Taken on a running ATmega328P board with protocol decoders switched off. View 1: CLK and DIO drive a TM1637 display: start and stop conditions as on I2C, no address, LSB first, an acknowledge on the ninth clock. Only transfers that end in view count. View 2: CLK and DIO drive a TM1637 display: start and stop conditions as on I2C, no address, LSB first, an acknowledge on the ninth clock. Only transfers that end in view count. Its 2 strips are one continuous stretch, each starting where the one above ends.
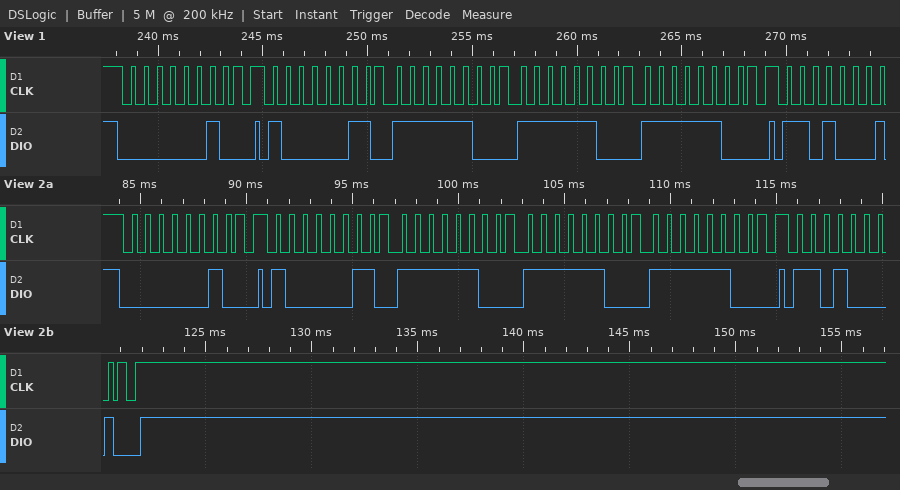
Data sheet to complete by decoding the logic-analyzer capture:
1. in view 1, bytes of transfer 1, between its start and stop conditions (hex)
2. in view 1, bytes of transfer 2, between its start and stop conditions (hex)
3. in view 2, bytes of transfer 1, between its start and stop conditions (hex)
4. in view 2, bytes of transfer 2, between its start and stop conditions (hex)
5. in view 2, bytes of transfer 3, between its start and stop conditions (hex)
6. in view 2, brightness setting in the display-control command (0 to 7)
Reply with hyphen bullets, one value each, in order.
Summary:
- 40
- C1 3F 3F 3F
- 40
- C1 3F 3F 3F
- 8B
- 3
